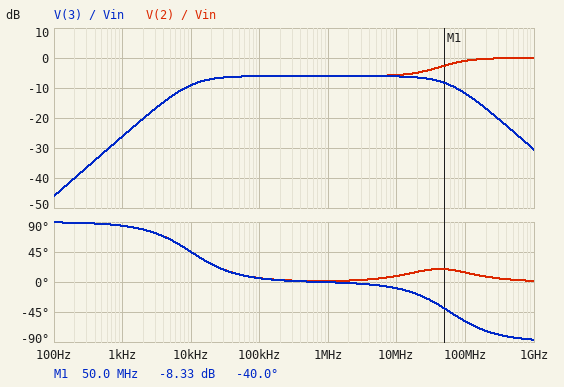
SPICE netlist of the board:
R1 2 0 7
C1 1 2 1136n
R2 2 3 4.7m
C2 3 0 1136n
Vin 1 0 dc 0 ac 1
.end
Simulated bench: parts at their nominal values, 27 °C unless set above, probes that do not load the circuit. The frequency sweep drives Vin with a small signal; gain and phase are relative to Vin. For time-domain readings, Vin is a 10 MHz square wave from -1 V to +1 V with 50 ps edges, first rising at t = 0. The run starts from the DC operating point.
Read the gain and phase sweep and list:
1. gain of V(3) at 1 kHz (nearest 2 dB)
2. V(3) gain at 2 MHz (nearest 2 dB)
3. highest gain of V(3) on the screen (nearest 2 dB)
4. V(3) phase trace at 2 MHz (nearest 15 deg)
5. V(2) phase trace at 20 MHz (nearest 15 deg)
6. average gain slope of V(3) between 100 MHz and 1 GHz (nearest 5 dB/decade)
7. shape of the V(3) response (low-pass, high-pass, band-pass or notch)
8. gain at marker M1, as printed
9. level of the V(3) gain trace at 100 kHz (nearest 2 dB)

-26 dB
-6 dB
-6 dB
0 deg
15 deg
-20 dB/decade
band-pass
-8.33 dB
-6 dB
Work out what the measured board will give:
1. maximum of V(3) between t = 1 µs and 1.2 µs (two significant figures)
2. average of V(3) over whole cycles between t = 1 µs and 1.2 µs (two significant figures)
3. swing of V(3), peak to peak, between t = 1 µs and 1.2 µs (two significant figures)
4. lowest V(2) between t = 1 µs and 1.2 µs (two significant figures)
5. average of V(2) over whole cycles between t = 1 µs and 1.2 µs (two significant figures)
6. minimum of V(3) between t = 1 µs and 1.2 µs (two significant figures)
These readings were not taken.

970 mV
470 mV
1.0 V
-1.0 V
470 mV
-36 mV
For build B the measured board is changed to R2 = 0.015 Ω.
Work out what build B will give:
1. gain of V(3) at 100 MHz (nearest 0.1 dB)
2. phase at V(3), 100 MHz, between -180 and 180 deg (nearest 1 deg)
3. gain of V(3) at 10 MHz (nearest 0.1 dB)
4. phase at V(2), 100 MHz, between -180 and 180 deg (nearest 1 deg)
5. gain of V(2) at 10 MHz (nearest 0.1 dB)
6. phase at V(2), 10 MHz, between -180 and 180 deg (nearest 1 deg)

-20.7 dB
-79 deg
-7.1 dB
5 deg
-3.8 dB
19 deg
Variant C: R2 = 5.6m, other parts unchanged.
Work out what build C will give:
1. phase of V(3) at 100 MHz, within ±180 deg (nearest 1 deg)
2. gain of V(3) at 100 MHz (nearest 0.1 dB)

-63 deg
-13.0 dB
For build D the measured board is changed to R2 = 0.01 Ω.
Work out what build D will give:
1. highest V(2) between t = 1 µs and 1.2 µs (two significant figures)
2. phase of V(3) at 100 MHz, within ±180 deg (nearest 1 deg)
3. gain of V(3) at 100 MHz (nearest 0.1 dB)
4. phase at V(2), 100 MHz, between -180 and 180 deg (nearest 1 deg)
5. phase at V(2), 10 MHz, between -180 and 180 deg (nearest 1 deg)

2.0 V
-74 deg
-17.4 dB
8 deg
16 deg
